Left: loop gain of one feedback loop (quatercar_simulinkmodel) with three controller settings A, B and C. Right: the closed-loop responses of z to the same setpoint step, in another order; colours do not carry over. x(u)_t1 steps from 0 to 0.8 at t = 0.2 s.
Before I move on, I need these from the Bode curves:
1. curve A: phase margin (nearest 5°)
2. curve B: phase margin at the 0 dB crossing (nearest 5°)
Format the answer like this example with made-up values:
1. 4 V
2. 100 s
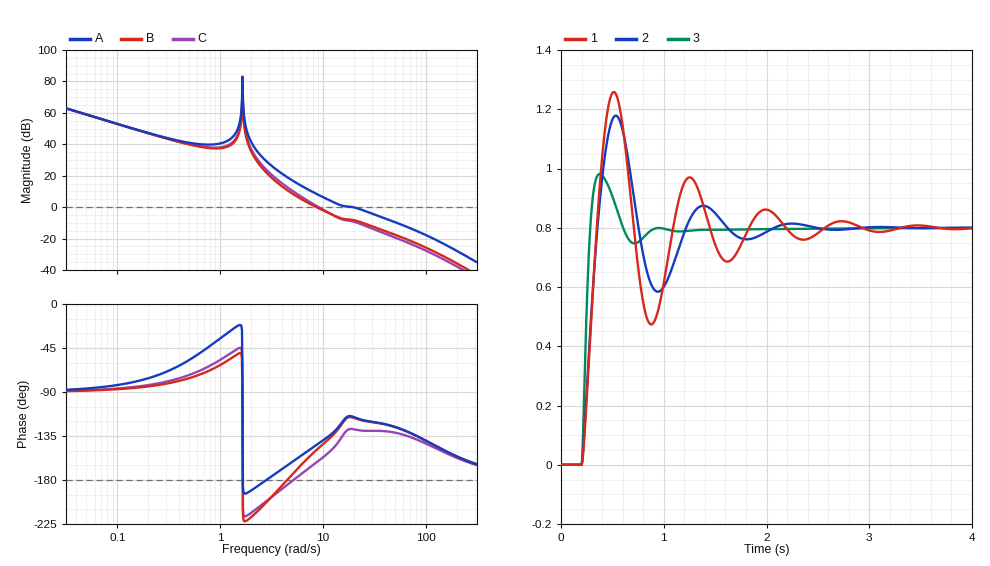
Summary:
1. 65°
2. 30°
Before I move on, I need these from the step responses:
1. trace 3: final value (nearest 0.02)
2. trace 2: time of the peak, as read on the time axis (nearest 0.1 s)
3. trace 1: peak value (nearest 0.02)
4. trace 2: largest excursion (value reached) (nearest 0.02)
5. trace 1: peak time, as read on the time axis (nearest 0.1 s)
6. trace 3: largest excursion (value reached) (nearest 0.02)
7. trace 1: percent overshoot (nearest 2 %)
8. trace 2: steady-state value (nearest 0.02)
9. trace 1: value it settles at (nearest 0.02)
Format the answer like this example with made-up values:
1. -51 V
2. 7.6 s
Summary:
1. 0.80
2. 0.5 s
3. 1.26
4. 1.18
5. 0.5 s
6. 0.98
7. 58 %
8. 0.80
9. 0.80
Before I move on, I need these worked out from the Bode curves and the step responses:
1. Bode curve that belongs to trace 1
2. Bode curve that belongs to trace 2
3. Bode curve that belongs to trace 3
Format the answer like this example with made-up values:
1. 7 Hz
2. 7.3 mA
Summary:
1. C
2. B
3. A
